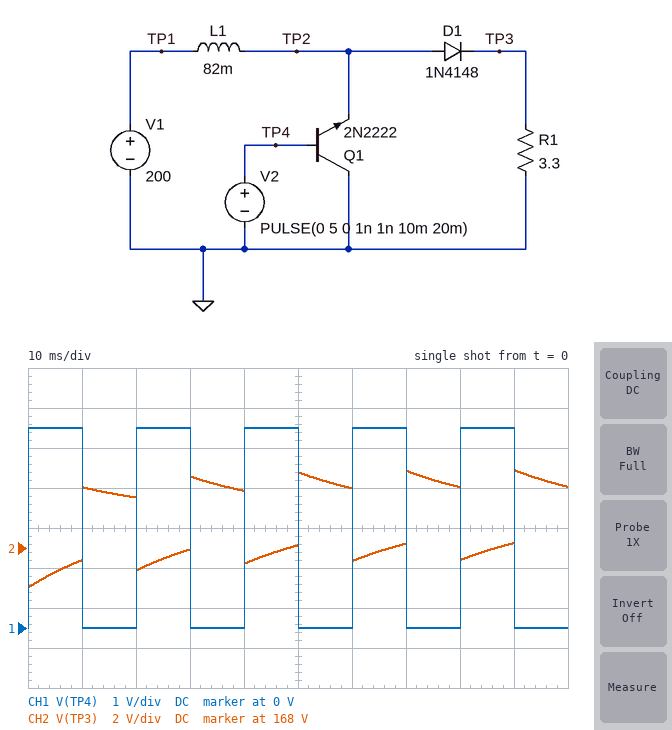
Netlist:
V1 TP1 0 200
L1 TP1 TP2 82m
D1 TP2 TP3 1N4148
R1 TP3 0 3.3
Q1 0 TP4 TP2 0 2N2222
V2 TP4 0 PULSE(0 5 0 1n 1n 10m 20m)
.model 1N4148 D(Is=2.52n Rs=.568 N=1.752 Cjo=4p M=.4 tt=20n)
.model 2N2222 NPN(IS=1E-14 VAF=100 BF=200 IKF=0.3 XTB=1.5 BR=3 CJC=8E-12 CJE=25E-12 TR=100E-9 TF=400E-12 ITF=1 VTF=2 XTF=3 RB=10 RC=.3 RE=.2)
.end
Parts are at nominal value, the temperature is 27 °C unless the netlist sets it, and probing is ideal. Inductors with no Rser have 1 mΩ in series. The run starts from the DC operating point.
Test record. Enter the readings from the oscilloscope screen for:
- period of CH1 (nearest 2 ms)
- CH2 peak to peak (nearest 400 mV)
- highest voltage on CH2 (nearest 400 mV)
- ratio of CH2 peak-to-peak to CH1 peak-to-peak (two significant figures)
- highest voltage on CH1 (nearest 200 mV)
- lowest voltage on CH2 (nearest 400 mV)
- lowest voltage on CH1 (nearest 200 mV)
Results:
20 ms
6.0 V
172.0 V
1.2
5.0 V
166.0 V
0 V
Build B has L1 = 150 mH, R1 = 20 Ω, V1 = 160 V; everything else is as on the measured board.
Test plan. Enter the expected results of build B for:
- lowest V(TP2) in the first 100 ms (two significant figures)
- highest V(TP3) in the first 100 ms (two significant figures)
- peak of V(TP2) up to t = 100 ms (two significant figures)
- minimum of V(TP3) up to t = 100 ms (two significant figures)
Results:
140 V
170 V
180 V
130 V
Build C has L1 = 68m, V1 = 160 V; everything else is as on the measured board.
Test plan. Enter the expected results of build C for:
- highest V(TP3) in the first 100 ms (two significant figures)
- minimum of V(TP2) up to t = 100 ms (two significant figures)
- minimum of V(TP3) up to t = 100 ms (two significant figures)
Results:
140 V
160 V
130 V
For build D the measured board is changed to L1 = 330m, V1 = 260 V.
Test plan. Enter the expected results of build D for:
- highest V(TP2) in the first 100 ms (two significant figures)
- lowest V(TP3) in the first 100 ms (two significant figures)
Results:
260 V
220 V
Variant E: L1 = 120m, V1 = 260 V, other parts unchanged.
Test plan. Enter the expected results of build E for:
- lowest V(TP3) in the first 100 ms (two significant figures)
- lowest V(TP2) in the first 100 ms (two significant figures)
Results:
220 V
260 V
